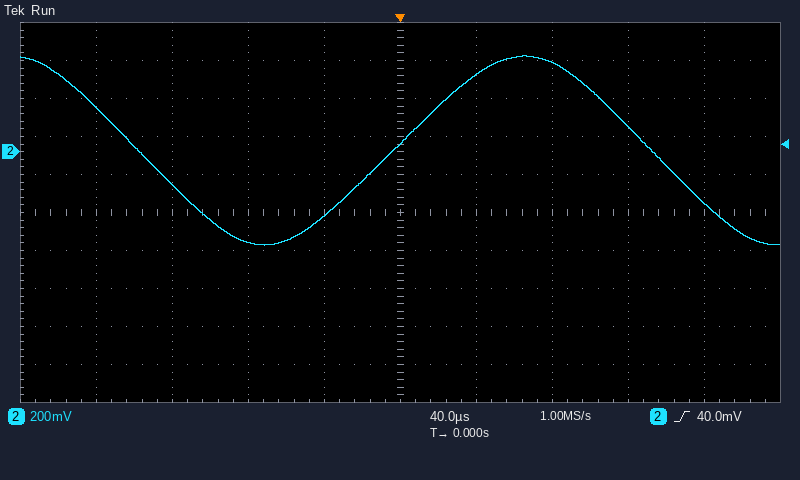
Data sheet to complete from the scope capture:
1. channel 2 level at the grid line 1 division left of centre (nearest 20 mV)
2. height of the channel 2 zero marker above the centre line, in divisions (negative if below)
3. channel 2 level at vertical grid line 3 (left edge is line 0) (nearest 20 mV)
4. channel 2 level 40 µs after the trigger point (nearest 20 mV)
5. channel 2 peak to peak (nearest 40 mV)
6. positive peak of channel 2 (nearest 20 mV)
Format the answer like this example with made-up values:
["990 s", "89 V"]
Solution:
["-340 mV", "+1.6 div", "-480 mV", "400 mV", "1.00 V", "500 mV"]
